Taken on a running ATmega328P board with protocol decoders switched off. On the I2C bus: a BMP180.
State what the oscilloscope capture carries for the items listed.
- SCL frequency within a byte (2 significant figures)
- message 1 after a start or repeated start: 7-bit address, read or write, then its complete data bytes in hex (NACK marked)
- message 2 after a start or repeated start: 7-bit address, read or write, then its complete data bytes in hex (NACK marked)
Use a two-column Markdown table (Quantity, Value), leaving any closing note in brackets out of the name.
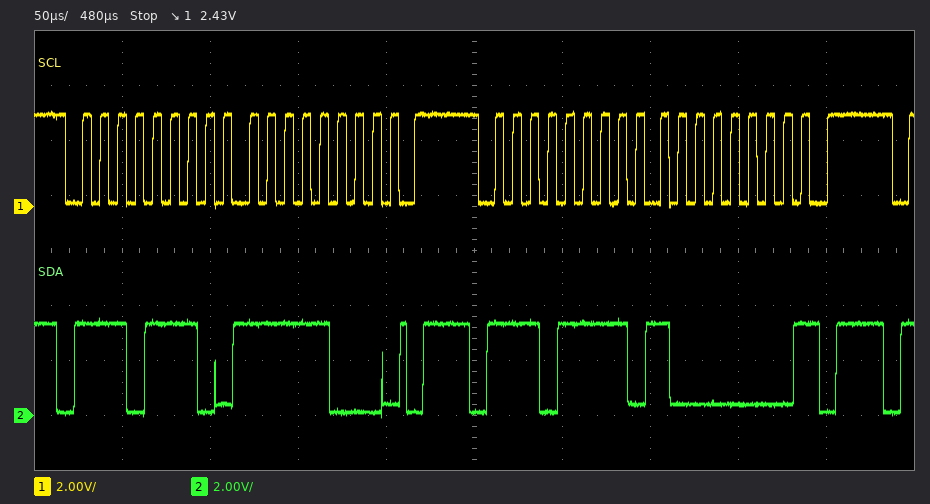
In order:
| Quantity | Value |
|---|---|
| SCL frequency within a byte | 100 kHz |
| message 1 after a start or repeated start: 7-bit address, read or write, then its complete data bytes in hex | 0x77 write: F8 |
| message 2 after a start or repeated start: 7-bit address, read or write, then its complete data bytes in hex | 0x77 read: 80 NACK |
